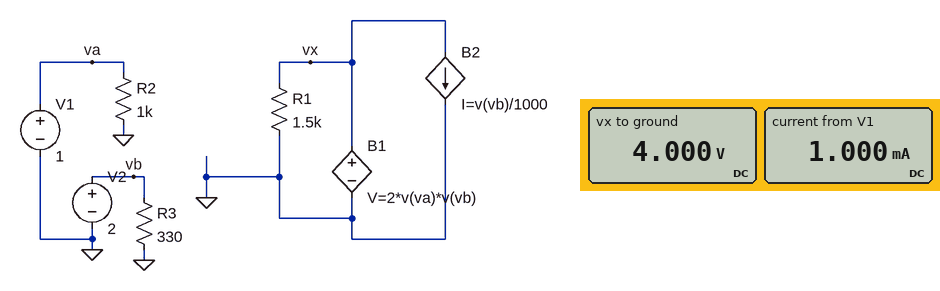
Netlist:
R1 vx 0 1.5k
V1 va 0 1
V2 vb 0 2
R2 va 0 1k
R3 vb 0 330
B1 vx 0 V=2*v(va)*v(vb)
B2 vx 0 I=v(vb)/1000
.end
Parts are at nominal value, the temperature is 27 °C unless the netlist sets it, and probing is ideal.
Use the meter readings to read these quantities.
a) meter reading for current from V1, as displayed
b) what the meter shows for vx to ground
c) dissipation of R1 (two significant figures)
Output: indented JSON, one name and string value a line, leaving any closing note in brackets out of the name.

{
  "meter reading for current from V1, as displayed": "1.000 mA",
  "what the meter shows for vx to ground": "4.000 V",
  "dissipation of R1": "11 mW"
}
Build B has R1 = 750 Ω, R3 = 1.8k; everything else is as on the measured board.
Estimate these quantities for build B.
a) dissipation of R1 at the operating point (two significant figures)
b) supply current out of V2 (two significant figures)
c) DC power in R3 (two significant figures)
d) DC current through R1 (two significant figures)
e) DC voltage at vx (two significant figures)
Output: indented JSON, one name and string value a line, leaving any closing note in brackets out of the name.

{
  "dissipation of R1 at the operating point": "21 mW",
  "supply current out of V2": "1.1 mA",
  "DC power in R3": "2.2 mW",
  "DC current through R1": "5.3 mA",
  "DC voltage at vx": "4.0 V"
}
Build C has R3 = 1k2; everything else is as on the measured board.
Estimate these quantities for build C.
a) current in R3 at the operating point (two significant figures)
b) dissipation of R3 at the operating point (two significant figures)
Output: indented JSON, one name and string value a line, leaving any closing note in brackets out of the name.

{
  "current in R3 at the operating point": "1.7 mA",
  "dissipation of R3 at the operating point": "3.3 mW"
}
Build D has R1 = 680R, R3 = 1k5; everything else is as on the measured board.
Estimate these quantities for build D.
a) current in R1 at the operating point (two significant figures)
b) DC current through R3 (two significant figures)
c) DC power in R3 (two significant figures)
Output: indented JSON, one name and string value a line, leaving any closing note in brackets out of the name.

{
  "current in R1 at the operating point": "5.9 mA",
  "DC current through R3": "1.3 mA",
  "DC power in R3": "2.7 mW"
}
